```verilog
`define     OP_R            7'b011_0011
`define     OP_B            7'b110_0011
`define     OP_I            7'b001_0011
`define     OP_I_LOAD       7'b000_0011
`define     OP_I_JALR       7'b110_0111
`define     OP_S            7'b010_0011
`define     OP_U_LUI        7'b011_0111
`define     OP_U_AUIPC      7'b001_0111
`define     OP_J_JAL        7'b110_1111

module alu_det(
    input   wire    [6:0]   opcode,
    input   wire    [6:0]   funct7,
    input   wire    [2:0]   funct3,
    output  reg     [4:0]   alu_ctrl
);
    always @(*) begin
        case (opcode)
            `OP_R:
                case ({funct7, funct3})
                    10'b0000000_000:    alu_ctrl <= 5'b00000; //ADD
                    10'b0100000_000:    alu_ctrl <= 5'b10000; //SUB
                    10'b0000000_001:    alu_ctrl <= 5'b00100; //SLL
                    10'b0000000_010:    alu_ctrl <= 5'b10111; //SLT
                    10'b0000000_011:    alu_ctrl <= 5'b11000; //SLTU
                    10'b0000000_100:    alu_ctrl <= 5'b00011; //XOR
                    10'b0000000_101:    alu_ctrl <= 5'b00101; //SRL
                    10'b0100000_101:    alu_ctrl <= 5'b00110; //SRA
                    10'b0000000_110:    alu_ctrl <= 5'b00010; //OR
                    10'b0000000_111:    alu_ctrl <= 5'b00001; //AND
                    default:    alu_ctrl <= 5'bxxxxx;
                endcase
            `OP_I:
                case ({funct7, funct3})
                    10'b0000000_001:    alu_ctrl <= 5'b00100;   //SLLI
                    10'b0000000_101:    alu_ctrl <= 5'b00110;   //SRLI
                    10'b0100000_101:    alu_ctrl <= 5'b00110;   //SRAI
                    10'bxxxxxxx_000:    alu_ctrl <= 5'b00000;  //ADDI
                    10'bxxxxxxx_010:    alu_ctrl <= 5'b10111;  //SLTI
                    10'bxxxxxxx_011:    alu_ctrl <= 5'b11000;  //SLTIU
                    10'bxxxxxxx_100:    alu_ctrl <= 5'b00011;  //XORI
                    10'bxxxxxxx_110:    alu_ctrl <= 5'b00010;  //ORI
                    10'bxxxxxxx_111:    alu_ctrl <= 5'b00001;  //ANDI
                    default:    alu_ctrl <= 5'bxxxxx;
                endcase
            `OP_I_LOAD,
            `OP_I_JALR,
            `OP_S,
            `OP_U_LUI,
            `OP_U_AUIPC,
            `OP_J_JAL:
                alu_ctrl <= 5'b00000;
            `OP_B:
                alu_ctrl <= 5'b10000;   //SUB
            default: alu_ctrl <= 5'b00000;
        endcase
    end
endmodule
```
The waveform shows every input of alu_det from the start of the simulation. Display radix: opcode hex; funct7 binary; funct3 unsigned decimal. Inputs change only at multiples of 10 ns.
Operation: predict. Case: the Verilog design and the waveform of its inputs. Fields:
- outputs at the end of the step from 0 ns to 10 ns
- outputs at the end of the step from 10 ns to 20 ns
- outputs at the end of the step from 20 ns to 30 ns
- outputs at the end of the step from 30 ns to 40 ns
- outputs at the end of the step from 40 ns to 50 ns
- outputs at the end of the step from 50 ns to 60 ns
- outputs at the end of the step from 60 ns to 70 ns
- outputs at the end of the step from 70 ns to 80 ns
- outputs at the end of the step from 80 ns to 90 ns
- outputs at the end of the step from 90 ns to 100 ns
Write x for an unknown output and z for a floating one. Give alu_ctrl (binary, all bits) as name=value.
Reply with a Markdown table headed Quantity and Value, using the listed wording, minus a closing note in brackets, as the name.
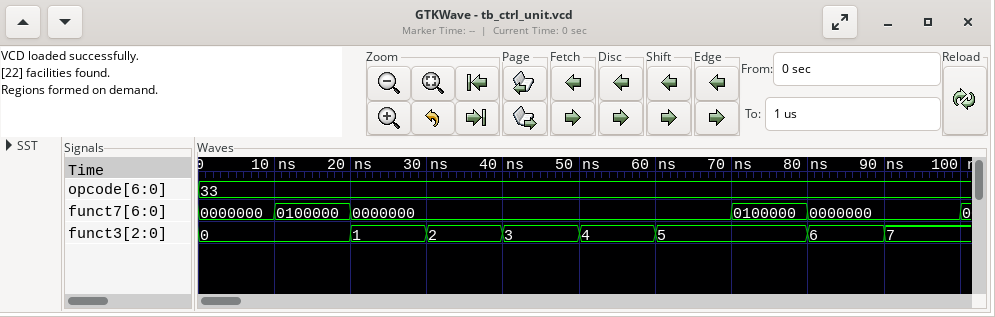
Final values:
| Quantity | Value |
|---|---|
| outputs at the end of the step from 0 ns to 10 ns | alu_ctrl=00000 |
| outputs at the end of the step from 10 ns to 20 ns | alu_ctrl=10000 |
| outputs at the end of the step from 20 ns to 30 ns | alu_ctrl=00100 |
| outputs at the end of the step from 30 ns to 40 ns | alu_ctrl=10111 |
| outputs at the end of the step from 40 ns to 50 ns | alu_ctrl=11000 |
| outputs at the end of the step from 50 ns to 60 ns | alu_ctrl=00011 |
| outputs at the end of the step from 60 ns to 70 ns | alu_ctrl=00101 |
| outputs at the end of the step from 70 ns to 80 ns | alu_ctrl=00110 |
| outputs at the end of the step from 80 ns to 90 ns | alu_ctrl=00010 |
| outputs at the end of the step from 90 ns to 100 ns | alu_ctrl=00001 |
